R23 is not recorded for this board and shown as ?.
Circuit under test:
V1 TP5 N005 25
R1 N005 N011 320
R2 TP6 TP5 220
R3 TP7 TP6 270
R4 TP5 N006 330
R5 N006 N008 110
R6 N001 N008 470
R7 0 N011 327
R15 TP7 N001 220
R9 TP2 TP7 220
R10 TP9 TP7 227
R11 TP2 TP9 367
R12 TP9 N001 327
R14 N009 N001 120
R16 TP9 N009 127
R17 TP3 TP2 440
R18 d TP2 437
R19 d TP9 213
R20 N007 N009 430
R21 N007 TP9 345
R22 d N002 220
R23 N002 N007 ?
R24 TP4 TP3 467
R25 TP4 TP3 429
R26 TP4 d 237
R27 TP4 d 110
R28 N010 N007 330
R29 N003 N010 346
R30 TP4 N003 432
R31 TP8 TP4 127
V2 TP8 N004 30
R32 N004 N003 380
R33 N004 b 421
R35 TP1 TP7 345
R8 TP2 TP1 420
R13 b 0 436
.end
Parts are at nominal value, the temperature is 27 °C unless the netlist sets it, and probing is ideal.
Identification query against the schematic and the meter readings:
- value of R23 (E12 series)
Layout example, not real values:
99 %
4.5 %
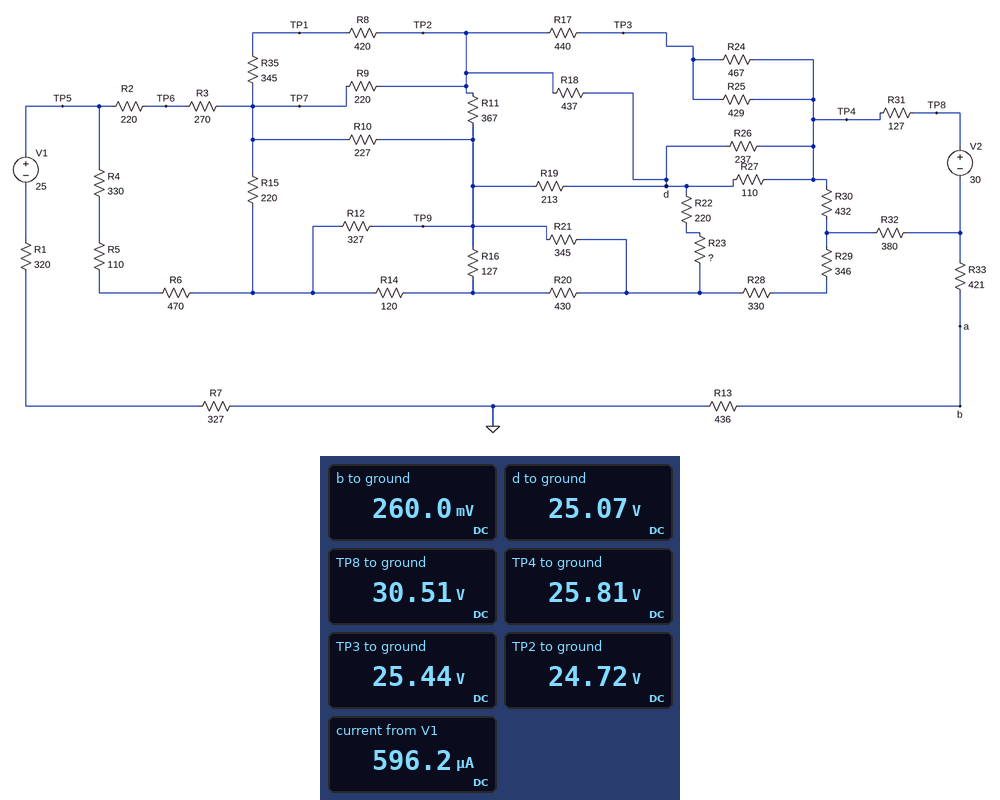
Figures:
150 Ω
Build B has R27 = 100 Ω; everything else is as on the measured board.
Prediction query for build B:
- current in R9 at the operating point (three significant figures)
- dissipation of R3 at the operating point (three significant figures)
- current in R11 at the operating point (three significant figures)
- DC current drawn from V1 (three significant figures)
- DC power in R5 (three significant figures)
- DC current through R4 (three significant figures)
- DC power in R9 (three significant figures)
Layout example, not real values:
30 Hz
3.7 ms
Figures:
1.04 mA
15.9 µW
1.07 mA
581 µA
12.6 µW
339 µA
239 µW
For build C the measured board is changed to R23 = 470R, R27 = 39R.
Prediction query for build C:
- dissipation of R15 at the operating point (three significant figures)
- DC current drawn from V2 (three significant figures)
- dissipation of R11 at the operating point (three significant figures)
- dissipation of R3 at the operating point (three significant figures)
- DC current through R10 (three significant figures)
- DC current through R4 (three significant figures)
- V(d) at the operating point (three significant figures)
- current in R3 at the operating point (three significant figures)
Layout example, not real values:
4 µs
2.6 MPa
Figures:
218 µW
37.0 mA
513 µW
9.34 µW
743 µA
341 µA
25.4 V
186 µA
